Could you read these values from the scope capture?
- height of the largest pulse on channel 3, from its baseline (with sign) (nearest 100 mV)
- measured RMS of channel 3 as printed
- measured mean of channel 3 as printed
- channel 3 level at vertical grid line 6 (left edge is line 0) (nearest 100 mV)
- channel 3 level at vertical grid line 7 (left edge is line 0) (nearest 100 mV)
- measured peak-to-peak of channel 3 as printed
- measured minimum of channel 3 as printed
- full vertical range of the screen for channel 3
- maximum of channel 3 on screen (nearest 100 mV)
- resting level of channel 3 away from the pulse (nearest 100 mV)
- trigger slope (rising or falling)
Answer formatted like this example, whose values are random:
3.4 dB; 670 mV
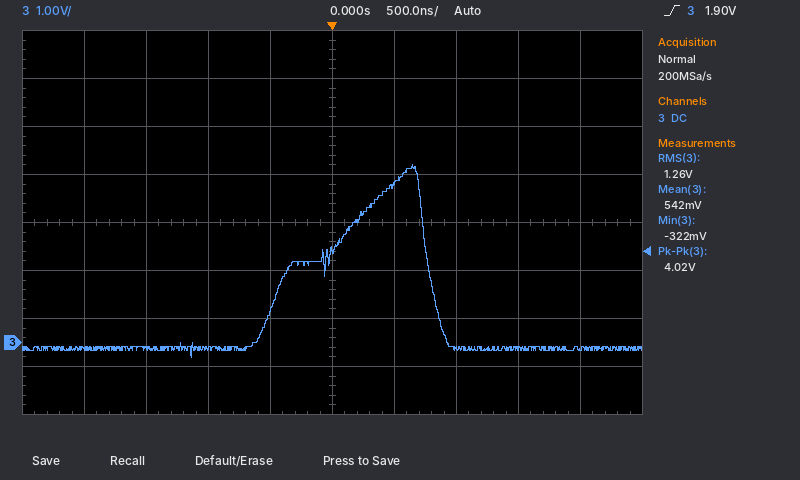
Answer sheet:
+3.8 V; 1.26 V; 542 mV; 3.3 V; -100 mV; 4.02 V; -322 mV; 8 V; 3.7 V; -100 mV; rising
